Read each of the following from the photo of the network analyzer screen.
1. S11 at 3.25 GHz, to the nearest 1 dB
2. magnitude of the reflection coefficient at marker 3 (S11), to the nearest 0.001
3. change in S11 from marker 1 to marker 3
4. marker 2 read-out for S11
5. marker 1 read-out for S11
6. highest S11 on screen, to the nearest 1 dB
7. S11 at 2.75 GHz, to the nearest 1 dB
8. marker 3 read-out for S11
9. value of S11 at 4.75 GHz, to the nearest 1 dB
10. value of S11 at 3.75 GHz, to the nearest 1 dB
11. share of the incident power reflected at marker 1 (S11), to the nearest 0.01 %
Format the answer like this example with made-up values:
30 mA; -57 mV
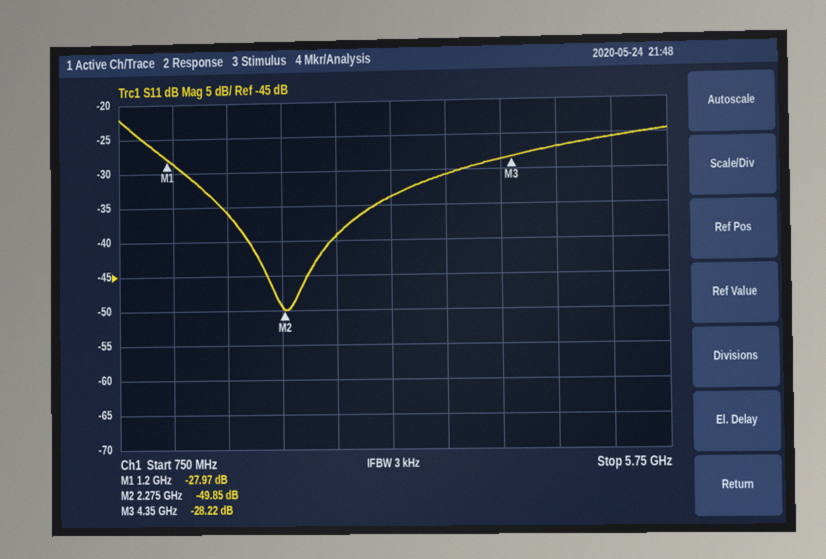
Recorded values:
-34 dB; 0.039; -0.25 dB; -49.85 dB; -27.97 dB; -22 dB; -39 dB; -28.22 dB; -27 dB; -31 dB; 0.16 %
